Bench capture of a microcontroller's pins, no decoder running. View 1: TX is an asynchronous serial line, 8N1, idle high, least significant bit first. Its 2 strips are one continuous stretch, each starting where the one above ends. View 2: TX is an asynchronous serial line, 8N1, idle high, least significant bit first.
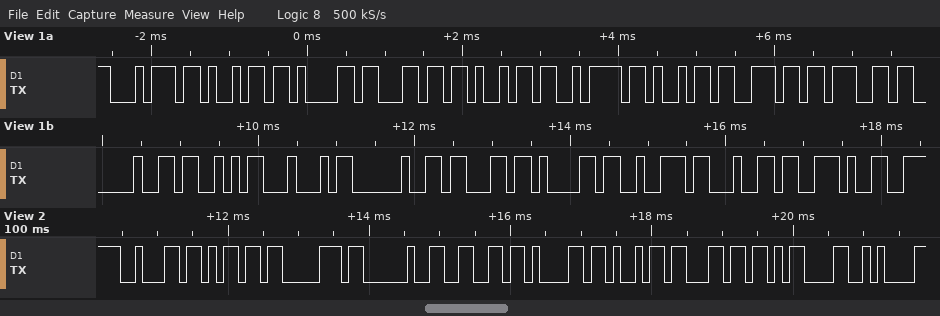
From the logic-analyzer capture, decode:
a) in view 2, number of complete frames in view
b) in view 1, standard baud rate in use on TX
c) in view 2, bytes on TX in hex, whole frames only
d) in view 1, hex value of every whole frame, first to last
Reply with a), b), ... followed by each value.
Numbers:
a) 10
b) 9600 baud
c) 0x62 0x6D 0x70 0x20 0x66 0x61 0x69 0x6C 0x0D 0x0A
d) 0x74 0x69 0x61 0x6C 0x69 0x7A 0x69 0x6E 0x67 0x20 0x53 0x44 0x20 0x63 0x61 0x72 0x64 0x2E
